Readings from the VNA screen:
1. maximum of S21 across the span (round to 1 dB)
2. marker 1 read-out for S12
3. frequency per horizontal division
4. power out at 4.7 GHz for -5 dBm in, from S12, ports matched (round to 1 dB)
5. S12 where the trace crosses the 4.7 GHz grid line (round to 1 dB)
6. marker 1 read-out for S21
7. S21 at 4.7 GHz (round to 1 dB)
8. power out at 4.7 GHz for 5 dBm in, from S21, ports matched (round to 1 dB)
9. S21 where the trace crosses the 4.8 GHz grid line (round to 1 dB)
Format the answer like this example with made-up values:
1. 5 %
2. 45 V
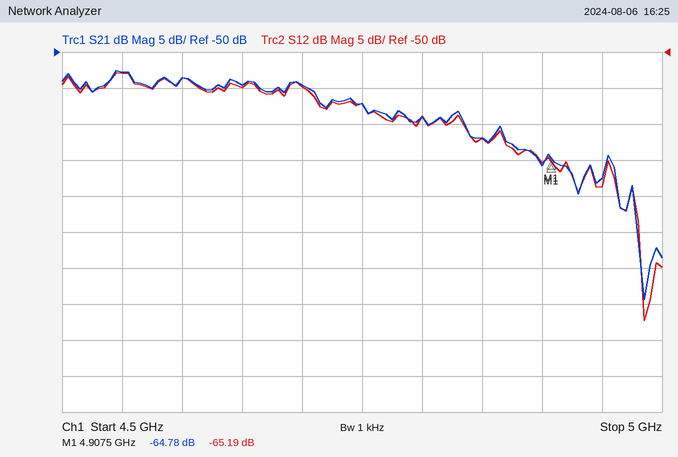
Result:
1. -53 dB
2. -65.19 dB
3. 50 MHz
4. -60 dBm
5. -55 dB
6. -64.78 dB
7. -55 dB
8. -50 dBm
9. -59 dB
